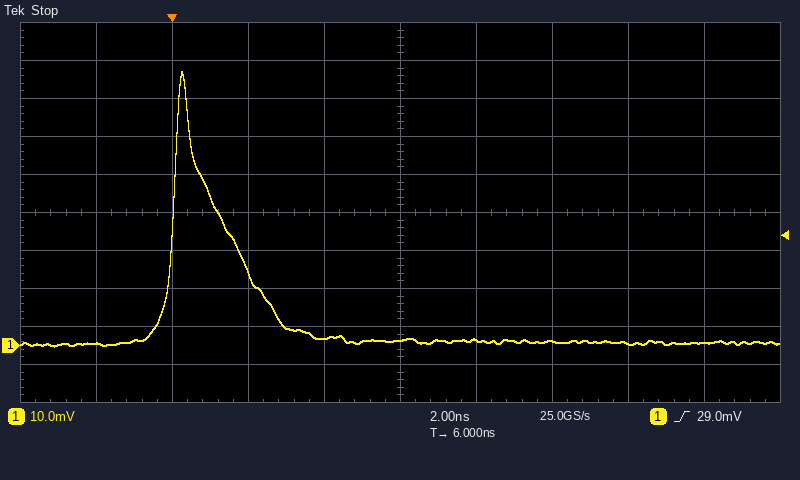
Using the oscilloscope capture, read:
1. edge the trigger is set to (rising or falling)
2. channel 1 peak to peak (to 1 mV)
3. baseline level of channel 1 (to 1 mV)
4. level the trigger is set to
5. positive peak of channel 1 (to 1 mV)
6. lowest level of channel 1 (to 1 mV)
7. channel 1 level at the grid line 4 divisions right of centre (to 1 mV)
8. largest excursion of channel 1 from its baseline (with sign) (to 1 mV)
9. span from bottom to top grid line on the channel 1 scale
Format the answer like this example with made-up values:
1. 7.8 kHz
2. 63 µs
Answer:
1. rising
2. 72 mV
3. 1 mV
4. 29.0 mV
5. 72 mV
6. 0 mV
7. 1 mV
8. +71 mV
9. 100 mV
